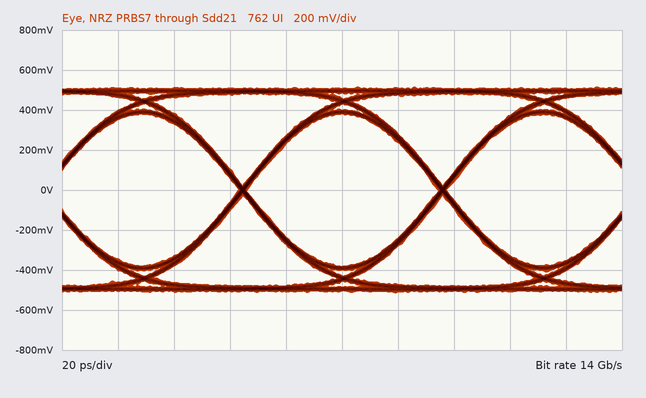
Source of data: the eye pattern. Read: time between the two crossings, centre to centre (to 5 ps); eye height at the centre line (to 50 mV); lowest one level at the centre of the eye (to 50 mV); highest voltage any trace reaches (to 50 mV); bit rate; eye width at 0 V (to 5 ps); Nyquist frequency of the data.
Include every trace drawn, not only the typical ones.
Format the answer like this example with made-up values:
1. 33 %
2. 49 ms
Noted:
1. 70 ps
2. 750 mV
3. 400 mV
4. 500 mV
5. 14 Gb/s
6. 70 ps
7. 7 GHz
